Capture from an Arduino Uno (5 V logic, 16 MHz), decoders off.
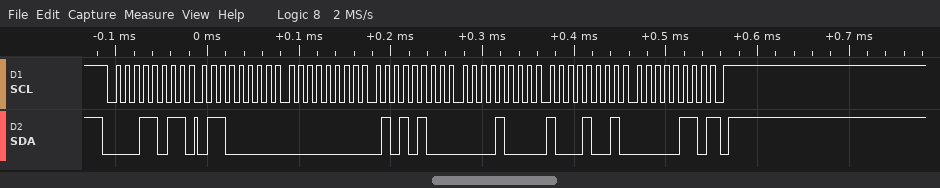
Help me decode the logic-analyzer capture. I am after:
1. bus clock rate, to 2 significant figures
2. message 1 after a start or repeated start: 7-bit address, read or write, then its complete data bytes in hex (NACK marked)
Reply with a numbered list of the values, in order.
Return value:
1. 100 kHz
2. 0x0D read: 60 00 54 08 89 06 NACK
